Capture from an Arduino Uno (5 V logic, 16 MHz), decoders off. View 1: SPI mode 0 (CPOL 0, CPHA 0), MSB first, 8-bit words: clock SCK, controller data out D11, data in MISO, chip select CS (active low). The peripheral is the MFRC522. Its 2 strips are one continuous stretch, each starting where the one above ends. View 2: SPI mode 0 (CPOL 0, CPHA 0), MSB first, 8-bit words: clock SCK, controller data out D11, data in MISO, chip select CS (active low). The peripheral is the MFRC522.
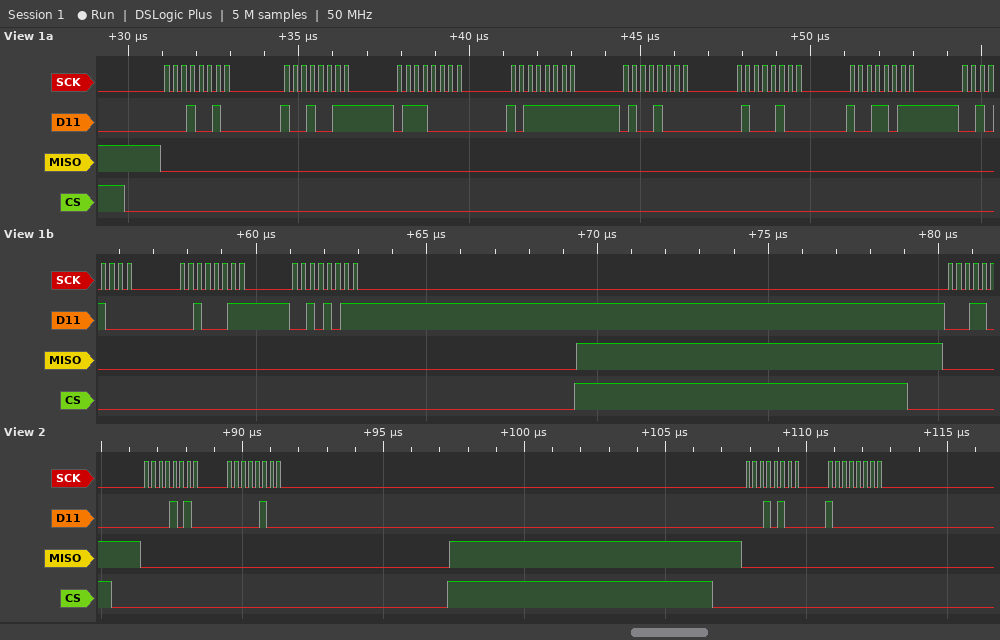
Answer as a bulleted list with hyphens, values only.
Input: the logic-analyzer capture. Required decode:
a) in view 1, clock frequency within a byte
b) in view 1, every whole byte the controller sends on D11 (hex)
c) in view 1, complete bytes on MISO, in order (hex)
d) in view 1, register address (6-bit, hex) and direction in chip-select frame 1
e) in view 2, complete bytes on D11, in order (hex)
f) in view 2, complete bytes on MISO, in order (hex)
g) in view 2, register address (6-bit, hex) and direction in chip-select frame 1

- 4 MHz
- 0x12 0x93 0x70 0xBF 0x48 0x44 0x9B 0x28 0x23 0x2B
- 0x00 0x00 0x00 0x00 0x00 0x00 0x00 0x00 0x00 0x00
- 0x09 write
- 0x0A 0x04 0x14 0x80
- 0x00 0x00 0x00 0x00
- 0x05 write
